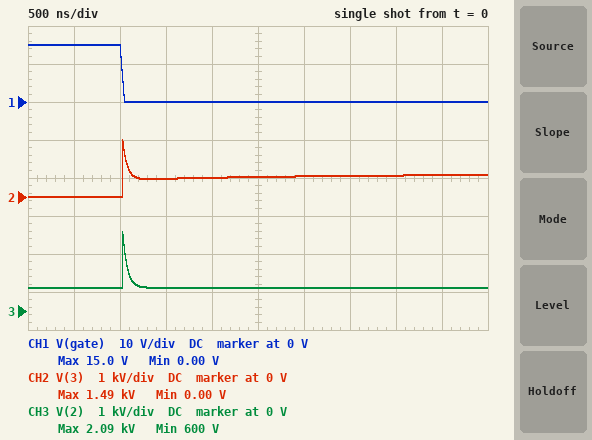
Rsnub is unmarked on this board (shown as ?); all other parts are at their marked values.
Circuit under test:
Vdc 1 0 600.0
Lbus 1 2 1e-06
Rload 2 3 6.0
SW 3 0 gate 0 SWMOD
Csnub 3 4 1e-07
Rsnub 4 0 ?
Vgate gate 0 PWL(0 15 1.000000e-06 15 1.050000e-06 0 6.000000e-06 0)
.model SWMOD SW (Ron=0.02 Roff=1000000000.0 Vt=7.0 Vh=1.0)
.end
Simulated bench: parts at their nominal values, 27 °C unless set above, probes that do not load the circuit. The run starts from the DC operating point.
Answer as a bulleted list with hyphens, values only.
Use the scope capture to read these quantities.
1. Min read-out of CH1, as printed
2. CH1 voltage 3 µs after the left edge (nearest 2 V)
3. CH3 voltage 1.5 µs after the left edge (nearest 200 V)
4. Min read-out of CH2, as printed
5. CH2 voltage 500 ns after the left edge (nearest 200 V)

- 0.00 V
- 0 V
- 600 V
- 0.00 V
- 0 V
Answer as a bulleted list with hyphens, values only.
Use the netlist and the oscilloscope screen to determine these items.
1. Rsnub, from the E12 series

- 15 Ω
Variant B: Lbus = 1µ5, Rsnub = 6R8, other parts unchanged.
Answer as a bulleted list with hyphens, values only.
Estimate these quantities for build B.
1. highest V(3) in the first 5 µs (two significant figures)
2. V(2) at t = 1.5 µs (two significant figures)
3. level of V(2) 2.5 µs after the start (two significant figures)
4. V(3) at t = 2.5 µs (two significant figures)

- 680 V
- 660 V
- 620 V
- 540 V
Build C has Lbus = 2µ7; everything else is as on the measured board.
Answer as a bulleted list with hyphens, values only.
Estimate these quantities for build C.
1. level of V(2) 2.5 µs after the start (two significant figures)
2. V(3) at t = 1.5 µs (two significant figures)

- 620 V
- 540 V
